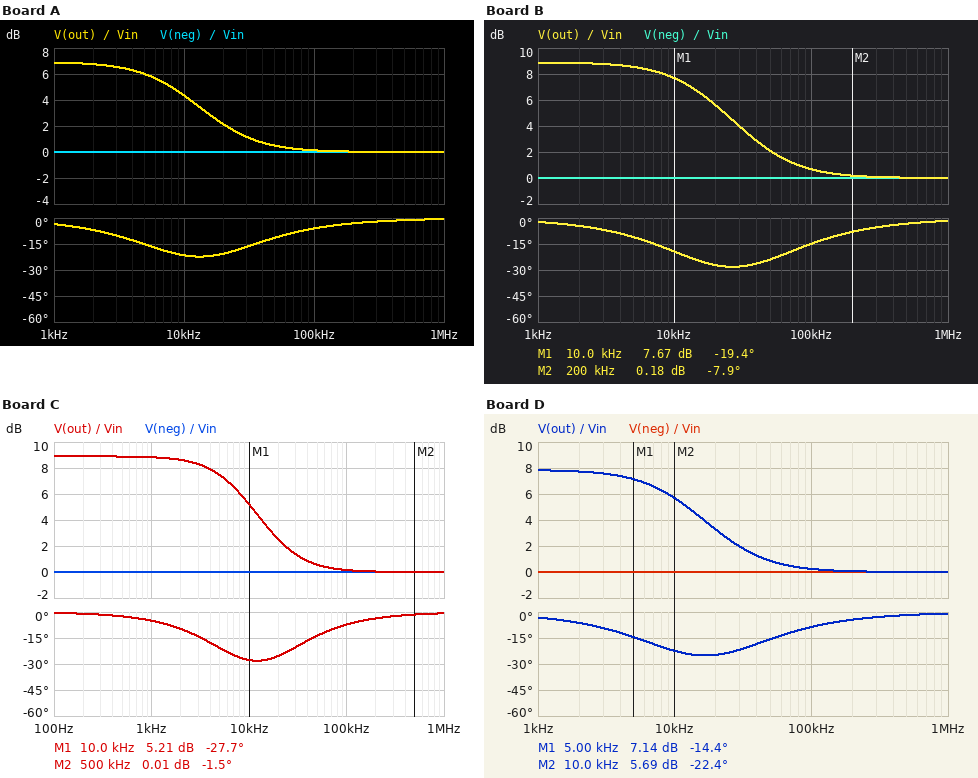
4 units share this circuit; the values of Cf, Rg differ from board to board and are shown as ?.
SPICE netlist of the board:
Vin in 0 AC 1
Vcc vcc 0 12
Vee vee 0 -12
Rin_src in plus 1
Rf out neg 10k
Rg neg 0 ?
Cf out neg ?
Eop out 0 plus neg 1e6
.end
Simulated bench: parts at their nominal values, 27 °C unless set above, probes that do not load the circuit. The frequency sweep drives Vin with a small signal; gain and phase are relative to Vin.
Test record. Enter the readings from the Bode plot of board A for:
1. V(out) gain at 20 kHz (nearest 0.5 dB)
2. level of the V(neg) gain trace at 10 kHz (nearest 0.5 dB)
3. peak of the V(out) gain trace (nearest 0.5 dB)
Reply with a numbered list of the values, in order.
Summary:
1. 2.0 dB
2. 0 dB
3. 7.0 dB
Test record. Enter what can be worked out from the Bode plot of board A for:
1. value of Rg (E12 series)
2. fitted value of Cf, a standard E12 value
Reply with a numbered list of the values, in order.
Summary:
1. 8.2 kΩ
2. 1.8 nF
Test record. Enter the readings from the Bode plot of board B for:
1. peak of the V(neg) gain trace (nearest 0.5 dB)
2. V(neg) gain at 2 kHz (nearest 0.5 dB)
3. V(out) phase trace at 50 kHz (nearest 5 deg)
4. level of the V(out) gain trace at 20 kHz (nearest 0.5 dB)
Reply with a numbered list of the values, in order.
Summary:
1. 0 dB
2. 0 dB
3. -25 deg
4. 5.5 dB
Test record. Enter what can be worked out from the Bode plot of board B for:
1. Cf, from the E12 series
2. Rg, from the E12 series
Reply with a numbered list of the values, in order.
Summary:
1. 1 nF
2. 5.6 kΩ
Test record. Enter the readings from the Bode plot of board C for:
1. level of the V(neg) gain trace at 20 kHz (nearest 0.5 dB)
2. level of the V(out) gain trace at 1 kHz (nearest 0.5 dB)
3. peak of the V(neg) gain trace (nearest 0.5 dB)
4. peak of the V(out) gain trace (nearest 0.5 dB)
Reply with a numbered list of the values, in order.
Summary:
1. 0 dB
2. 9.0 dB
3. 0 dB
4. 9.0 dB
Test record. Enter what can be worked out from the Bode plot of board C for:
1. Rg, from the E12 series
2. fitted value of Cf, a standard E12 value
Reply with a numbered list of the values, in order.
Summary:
1. 5.6 kΩ
2. 2.2 nF
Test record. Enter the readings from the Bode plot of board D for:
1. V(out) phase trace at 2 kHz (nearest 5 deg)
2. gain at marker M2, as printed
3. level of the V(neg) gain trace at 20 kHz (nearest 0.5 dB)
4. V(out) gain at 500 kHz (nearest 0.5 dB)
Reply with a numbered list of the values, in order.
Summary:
1. -5 deg
2. 5.69 dB
3. 0 dB
4. 0 dB
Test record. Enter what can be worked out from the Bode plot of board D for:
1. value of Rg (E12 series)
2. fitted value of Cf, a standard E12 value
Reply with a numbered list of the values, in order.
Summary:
1. 6.8 kΩ
2. 1.5 nF
